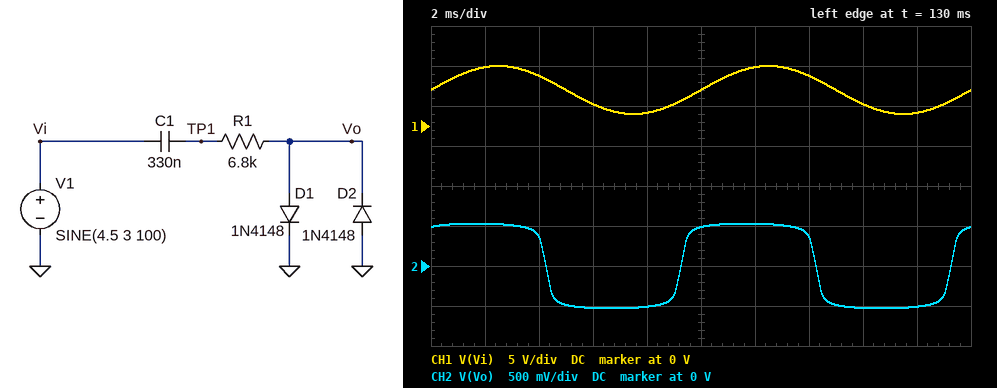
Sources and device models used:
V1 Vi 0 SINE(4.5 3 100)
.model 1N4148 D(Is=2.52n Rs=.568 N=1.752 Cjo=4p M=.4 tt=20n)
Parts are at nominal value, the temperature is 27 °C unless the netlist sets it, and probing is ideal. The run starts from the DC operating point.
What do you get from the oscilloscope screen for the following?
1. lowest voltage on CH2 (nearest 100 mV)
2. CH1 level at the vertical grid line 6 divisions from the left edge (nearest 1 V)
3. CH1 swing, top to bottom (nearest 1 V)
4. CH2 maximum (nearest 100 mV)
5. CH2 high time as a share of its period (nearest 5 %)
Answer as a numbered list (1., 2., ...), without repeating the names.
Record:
1. -500 mV
2. 7 V
3. 6 V
4. 500 mV
5. 50 %
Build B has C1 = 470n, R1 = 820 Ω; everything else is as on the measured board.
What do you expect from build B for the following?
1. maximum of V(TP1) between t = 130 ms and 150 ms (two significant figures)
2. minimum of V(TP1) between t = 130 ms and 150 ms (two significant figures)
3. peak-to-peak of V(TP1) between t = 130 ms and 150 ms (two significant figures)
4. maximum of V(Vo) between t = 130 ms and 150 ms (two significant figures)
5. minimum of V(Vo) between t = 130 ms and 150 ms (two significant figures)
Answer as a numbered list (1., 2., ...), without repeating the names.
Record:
1. 1.3 V
2. -1.3 V
3. 2.5 V
4. 580 mV
5. -580 mV
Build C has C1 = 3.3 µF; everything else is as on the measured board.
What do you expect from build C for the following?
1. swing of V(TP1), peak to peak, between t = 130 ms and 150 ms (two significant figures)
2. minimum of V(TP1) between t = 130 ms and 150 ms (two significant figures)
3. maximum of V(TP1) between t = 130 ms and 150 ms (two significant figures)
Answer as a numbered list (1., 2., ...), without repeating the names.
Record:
1. 6.0 V
2. -3.0 V
3. 3.0 V
